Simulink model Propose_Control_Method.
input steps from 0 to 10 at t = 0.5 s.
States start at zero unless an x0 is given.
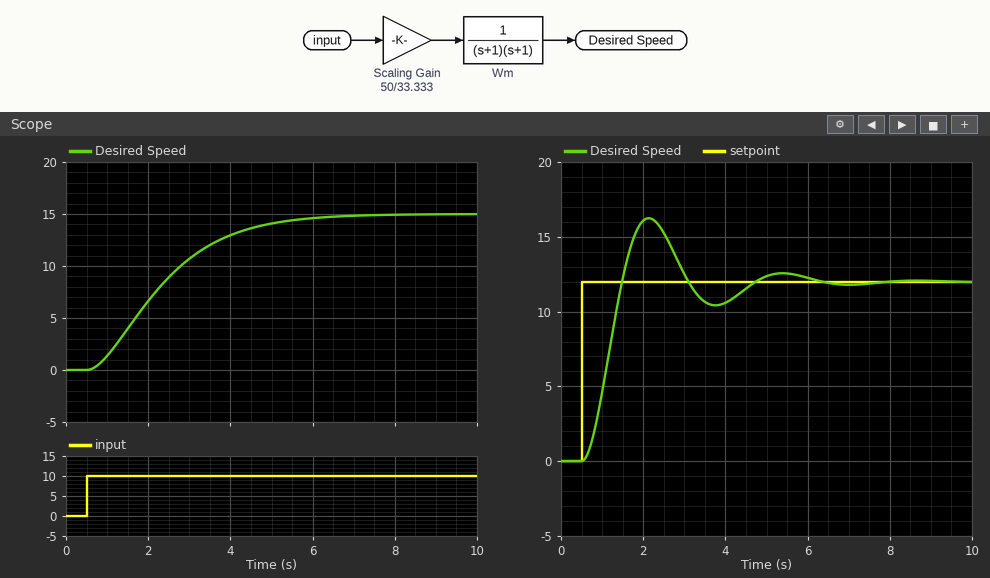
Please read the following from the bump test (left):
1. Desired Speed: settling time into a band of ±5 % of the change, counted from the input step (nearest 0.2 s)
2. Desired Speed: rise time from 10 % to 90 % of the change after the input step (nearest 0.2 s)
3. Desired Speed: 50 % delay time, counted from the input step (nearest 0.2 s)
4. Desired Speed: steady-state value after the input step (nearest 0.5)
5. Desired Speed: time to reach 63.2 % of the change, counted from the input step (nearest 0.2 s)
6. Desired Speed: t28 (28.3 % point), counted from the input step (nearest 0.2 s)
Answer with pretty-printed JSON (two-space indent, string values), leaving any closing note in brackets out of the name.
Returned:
{
  "Desired Speed: settling time into a band of ±5 % of the change, counted from the input step": "4.8 s",
  "Desired Speed: rise time from 10 % to 90 % of the change after the input step": "3.4 s",
  "Desired Speed: 50 % delay time, counted from the input step": "1.6 s",
  "Desired Speed: steady-state value after the input step": "15.0",
  "Desired Speed: time to reach 63.2 % of the change, counted from the input step": "2.2 s",
  "Desired Speed: t28 (28.3 % point), counted from the input step": "1.0 s"
}
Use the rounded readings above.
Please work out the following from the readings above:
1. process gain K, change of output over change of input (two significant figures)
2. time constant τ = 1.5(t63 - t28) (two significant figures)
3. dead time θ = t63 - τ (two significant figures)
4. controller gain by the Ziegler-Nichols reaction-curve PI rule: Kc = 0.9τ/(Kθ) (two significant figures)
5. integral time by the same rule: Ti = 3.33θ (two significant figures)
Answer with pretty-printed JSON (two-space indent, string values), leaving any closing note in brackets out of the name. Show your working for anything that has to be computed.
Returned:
{
  "process gain K, change of output over change of input": "(15 - 0) / 10 = 1.5",
  "time constant τ = 1.5(t63 - t28)": "1.5 × (2.2 - 1) = 1.8 s",
  "dead time θ = t63 - τ": "2.2 - 1.8 = 0.40 s",
  "controller gain by the Ziegler-Nichols reaction-curve PI rule: Kc = 0.9τ/(Kθ)": "0.9 × 1.8 / (1.5 × 0.4) = 2.7",
  "integral time by the same rule: Ti = 3.33θ": "3.33 × 0.4 = 1.3 s"
}
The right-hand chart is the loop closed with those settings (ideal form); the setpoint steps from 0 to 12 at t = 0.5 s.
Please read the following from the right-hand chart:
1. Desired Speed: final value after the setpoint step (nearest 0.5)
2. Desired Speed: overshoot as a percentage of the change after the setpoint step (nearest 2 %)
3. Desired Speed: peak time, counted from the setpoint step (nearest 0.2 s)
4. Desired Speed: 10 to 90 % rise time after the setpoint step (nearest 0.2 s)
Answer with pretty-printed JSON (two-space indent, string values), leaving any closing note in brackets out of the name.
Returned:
{
  "Desired Speed: final value after the setpoint step": "12.0",
  "Desired Speed: overshoot as a percentage of the change after the setpoint step": "36 %",
  "Desired Speed: peak time, counted from the setpoint step": "1.6 s",
  "Desired Speed: 10 to 90 % rise time after the setpoint step": "0.6 s"
}
